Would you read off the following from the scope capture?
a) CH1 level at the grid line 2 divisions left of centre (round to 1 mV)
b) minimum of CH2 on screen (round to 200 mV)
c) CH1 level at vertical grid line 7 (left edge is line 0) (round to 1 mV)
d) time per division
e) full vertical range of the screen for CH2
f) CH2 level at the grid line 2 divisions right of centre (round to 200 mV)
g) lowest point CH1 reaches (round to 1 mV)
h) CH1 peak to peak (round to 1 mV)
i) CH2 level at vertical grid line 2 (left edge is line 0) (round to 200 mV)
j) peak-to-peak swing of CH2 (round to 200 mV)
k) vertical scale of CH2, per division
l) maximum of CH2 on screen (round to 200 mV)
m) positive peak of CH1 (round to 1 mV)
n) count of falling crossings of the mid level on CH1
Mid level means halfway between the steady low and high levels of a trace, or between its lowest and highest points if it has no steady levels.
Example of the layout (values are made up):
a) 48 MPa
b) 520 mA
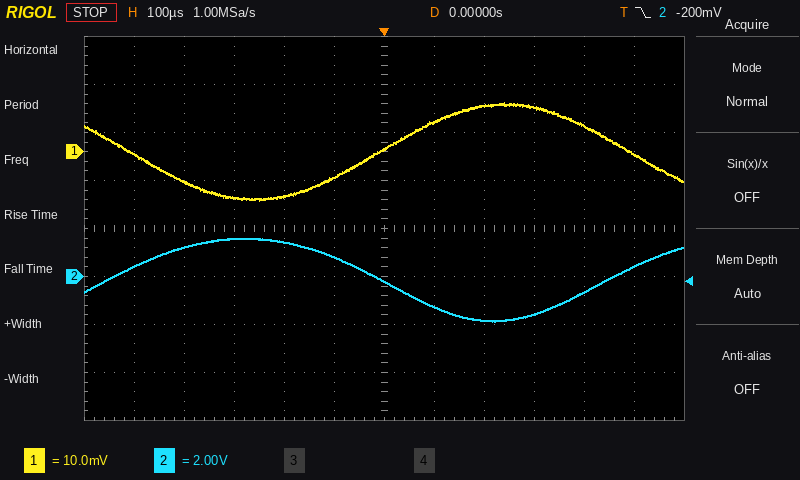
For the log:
a) -9 mV
b) -1.8 V
c) 6 mV
d) 100 µs
e) 16 V
f) -1.8 V
g) -10 mV
h) 20 mV
i) 1.2 V
j) 3.4 V
k) 2 V
l) 1.6 V
m) 10 mV
n) 2
